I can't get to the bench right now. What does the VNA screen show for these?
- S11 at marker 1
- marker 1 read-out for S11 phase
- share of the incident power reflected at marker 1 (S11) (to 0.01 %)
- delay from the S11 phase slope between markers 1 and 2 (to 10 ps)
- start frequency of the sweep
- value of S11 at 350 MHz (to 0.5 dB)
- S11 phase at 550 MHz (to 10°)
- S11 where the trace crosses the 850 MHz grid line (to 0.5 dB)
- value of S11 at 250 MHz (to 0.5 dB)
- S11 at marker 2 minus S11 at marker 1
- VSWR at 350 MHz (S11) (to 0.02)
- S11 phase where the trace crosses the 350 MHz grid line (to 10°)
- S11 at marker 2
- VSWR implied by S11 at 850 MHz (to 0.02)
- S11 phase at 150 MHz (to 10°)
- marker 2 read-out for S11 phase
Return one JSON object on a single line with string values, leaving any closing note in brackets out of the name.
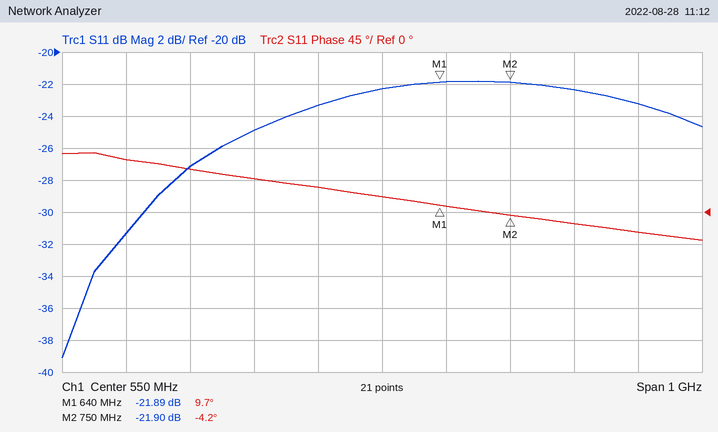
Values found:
{"S11 at marker 1": "-21.89 dB", "marker 1 read-out for S11 phase": "9.7°", "share of the incident power reflected at marker 1 (S11)": "0.65 %", "delay from the S11 phase slope between markers 1 and 2": "350 ps", "start frequency of the sweep": "50 MHz", "value of S11 at 350 MHz": "-25.0 dB", "S11 phase at 550 MHz": "20°", "S11 where the trace crosses the 850 MHz grid line": "-22.5 dB", "value of S11 at 250 MHz": "-27.0 dB", "S11 at marker 2 minus S11 at marker 1": "-0.01 dB", "VSWR at 350 MHz (S11)": "1.12", "S11 phase where the trace crosses the 350 MHz grid line": "50°", "S11 at marker 2": "-21.90 dB", "VSWR implied by S11 at 850 MHz": "1.16", "S11 phase at 150 MHz": "70°", "marker 2 read-out for S11 phase": "-4.2°"}
